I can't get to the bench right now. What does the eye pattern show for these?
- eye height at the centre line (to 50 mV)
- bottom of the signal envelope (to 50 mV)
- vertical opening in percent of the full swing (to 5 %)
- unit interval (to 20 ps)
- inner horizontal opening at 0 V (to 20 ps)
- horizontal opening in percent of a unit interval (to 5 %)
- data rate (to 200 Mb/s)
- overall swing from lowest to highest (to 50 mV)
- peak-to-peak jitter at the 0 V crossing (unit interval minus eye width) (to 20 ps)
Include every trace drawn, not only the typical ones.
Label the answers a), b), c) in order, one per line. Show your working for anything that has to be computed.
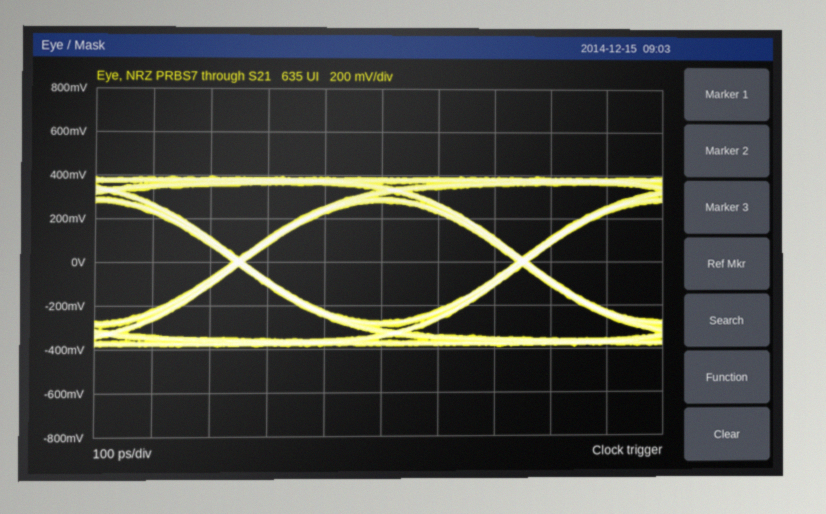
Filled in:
a) 550 mV
b) -400 mV
c) 550 mV / 800 mV ≈ 68.8 %, so 70 % to the nearest 5 %
d) 500 ps
e) 480 ps
f) 480 ps / 500 ps ≈ 96.0 %, so 95 % to the nearest 5 %
g) 2.0 Gb/s
h) 800 mV
i) 20 ps
